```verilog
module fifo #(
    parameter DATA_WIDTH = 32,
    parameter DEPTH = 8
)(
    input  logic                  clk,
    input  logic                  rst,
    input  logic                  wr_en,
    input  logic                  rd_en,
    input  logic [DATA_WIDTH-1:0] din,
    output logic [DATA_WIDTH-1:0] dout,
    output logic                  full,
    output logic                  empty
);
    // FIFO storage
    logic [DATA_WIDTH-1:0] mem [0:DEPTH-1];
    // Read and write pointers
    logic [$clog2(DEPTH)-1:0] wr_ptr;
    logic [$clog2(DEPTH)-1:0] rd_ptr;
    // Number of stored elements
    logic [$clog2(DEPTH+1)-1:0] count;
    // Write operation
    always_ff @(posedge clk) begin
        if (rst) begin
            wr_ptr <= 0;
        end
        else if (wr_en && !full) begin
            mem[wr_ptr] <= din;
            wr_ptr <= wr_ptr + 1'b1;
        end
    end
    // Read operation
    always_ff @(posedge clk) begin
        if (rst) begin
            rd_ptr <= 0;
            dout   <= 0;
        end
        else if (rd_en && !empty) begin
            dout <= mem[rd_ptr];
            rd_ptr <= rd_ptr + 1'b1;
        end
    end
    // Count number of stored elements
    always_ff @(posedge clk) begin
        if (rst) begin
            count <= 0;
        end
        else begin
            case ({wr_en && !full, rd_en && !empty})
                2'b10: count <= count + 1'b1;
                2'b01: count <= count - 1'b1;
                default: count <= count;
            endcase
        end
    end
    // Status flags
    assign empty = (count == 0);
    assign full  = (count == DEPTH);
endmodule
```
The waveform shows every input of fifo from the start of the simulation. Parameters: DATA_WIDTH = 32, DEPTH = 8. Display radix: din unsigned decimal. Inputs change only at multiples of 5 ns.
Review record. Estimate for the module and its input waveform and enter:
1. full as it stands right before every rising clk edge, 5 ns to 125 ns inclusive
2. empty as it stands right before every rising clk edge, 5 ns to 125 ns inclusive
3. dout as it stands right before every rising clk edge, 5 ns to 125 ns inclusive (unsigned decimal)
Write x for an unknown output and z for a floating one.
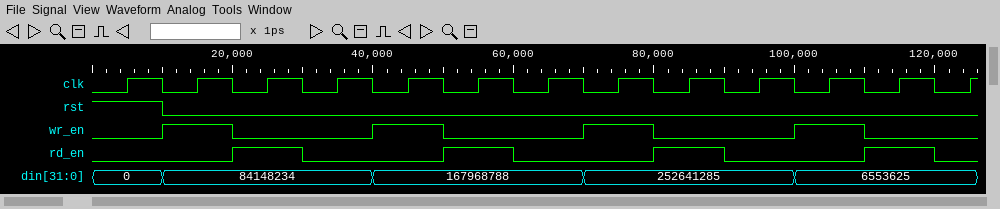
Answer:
x 0 0 0 0 0 0 0 0 0 0 0 0
x 1 0 1 1 0 1 1 0 1 1 0 1
x, 0, 0, 84148234, 84148234, 84148234, 167968788, 167968788, 167968788, 252641285, 252641285, 252641285, 6553625
